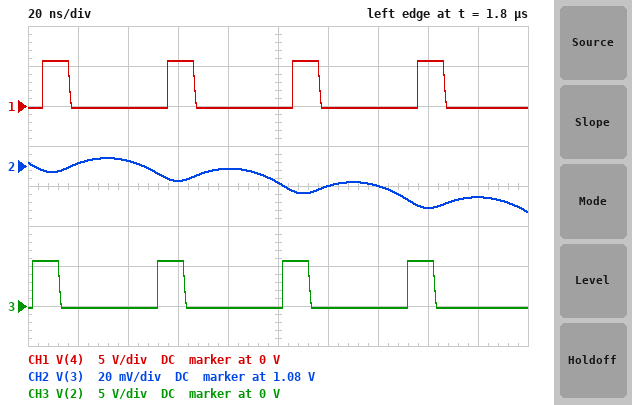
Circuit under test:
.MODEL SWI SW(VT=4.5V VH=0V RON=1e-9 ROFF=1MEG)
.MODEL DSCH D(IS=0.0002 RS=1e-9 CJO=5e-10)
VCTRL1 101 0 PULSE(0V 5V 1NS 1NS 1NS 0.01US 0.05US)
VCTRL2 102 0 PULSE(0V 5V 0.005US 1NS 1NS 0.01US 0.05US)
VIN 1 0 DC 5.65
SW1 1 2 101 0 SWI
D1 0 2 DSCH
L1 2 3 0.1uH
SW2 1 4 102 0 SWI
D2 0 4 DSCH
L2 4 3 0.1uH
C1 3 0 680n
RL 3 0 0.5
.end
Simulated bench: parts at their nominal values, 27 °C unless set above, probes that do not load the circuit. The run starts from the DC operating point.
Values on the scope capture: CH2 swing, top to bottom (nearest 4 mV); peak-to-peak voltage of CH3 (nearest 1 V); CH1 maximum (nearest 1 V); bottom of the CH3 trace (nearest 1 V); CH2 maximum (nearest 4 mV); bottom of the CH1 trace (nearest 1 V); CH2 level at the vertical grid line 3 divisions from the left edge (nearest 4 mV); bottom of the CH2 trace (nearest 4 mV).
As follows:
28 mV
6 V
6 V
0 V
1.084 V
0 V
1.072 V
1.056 V
